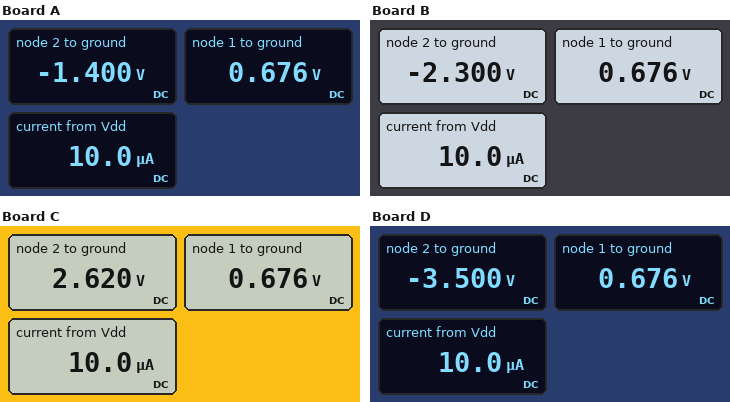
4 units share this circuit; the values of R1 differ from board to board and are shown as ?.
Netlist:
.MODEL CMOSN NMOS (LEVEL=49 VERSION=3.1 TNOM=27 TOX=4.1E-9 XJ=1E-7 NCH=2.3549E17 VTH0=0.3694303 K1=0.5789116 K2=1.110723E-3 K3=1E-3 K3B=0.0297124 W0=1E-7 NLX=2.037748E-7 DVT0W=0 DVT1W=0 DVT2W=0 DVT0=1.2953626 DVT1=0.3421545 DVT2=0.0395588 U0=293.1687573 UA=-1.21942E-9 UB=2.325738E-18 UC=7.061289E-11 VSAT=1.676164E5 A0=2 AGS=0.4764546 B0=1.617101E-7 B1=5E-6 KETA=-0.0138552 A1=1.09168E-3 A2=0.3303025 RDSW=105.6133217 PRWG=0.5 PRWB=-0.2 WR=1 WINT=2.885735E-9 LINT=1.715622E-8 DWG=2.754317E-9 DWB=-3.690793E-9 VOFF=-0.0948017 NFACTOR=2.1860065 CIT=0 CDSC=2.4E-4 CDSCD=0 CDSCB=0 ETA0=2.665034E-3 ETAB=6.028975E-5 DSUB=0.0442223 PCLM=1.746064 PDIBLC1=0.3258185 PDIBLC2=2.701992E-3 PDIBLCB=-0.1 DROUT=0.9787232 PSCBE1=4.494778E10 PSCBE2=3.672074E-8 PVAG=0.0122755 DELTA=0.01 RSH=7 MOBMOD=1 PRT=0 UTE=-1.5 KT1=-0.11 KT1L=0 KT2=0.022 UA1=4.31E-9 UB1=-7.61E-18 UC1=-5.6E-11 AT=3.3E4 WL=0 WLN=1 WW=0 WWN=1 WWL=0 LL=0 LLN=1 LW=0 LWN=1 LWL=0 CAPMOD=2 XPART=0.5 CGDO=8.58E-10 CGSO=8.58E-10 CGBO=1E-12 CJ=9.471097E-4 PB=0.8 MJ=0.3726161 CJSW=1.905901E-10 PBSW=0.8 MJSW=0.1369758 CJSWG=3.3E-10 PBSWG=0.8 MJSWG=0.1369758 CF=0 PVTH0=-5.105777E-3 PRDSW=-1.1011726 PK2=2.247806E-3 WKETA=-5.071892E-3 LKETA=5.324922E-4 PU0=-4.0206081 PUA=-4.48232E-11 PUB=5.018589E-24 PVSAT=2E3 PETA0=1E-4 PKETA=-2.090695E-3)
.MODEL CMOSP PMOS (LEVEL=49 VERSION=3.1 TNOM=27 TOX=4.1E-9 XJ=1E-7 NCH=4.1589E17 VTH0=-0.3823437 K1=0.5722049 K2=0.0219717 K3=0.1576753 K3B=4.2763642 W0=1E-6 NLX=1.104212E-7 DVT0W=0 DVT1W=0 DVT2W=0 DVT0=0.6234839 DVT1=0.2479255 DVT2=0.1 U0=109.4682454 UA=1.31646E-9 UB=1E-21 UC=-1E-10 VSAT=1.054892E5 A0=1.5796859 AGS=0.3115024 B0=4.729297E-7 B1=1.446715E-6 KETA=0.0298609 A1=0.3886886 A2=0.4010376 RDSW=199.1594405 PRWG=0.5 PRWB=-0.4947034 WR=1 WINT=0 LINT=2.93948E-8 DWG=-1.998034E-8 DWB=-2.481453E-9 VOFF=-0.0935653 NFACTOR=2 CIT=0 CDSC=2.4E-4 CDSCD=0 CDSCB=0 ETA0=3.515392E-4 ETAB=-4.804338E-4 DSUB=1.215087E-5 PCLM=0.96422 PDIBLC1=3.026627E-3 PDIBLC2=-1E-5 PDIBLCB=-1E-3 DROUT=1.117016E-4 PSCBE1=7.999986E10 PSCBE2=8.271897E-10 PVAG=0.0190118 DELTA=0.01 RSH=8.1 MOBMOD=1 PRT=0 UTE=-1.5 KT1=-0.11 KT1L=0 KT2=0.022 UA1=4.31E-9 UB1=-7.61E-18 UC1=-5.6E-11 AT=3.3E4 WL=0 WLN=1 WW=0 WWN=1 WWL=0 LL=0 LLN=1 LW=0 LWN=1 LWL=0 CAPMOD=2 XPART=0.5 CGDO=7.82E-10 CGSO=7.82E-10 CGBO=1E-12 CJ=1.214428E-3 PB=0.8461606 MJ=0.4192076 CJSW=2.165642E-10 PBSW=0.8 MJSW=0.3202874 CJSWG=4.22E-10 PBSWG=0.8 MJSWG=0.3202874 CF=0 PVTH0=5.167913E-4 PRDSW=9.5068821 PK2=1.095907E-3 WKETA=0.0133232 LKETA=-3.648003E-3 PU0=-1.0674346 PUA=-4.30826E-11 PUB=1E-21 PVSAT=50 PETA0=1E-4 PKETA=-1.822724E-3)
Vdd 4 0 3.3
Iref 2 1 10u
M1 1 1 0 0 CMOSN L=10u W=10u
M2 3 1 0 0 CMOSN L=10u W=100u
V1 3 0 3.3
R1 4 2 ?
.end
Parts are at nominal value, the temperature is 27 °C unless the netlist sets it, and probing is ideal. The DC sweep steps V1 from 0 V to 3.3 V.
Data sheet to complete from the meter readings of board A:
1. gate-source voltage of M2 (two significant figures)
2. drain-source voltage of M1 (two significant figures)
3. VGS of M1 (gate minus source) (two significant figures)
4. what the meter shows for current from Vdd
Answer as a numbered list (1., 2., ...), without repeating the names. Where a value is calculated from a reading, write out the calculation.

1. 676 mV = 680 mV
2. 676 mV = 680 mV
3. 676 mV = 680 mV
4. 10.0 µA
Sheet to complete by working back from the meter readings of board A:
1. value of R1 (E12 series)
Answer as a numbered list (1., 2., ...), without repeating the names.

1. 470 kΩ
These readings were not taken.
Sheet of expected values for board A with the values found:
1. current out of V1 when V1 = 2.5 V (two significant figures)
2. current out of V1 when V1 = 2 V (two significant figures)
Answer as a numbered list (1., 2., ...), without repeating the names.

1. 100 µA
2. 100 µA
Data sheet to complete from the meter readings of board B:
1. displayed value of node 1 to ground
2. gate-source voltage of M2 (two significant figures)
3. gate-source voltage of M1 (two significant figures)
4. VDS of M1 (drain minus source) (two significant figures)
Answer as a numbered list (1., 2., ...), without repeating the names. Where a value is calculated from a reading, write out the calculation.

1. 0.676 V
2. 676 mV = 680 mV
3. 676 mV = 680 mV
4. 676 mV = 680 mV
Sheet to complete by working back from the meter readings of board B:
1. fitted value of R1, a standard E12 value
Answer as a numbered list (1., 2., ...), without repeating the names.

1. 560 kΩ
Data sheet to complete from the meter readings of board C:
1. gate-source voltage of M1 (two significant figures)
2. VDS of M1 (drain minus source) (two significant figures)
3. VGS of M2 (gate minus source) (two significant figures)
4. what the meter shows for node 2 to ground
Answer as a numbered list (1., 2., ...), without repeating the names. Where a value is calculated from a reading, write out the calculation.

1. 676 mV = 680 mV
2. 676 mV = 680 mV
3. 676 mV = 680 mV
4. 2.620 V
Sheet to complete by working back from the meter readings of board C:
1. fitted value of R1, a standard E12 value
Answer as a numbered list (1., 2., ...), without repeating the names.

1. 68 kΩ
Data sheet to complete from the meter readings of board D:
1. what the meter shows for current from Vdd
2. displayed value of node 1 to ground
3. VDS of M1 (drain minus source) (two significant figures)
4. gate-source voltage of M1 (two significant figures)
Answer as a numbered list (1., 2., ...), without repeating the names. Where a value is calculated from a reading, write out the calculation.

1. 10.0 µA
2. 0.676 V
3. 676 mV = 680 mV
4. 676 mV = 680 mV
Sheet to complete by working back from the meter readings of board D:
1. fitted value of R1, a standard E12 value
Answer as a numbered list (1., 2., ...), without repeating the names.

1. 680 kΩ
